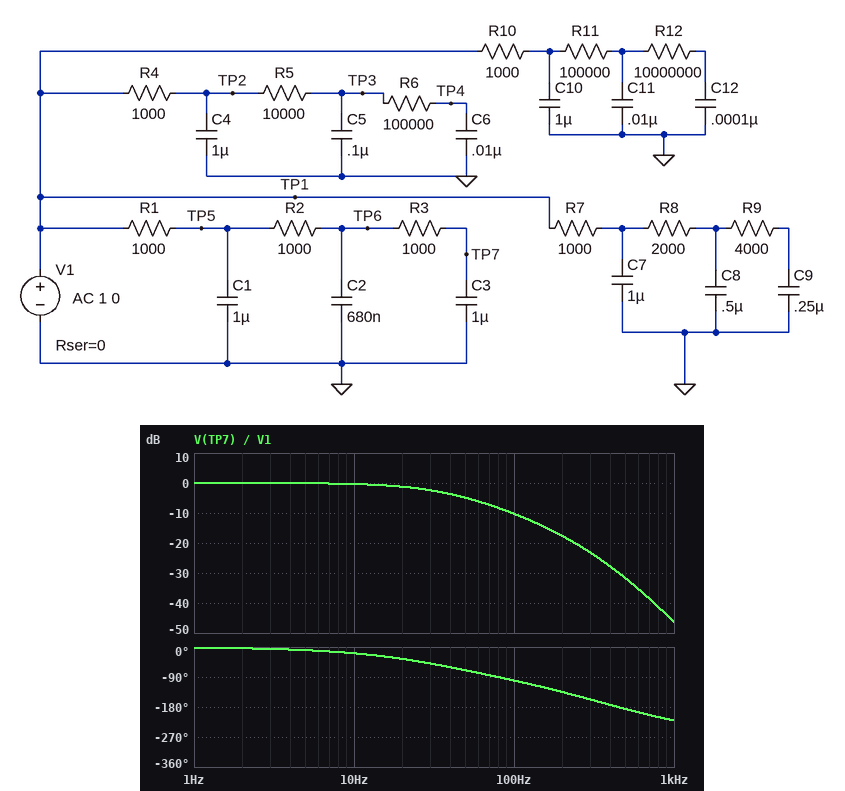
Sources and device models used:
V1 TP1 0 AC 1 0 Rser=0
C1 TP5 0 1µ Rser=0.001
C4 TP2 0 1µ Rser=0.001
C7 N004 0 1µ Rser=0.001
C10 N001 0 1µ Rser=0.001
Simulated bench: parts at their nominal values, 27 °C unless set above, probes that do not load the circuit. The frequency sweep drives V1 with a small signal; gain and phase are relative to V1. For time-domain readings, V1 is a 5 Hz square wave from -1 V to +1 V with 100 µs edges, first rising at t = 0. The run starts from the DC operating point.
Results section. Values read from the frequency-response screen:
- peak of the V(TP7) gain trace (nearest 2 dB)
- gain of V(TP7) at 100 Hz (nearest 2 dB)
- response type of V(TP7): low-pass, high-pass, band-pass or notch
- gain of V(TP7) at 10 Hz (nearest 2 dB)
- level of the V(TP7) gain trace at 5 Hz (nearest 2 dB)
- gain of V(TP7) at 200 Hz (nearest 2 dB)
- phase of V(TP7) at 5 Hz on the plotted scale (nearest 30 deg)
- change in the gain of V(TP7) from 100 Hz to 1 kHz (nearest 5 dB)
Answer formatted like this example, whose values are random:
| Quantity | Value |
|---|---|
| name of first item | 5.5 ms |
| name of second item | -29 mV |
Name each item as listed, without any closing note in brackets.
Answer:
| Quantity | Value |
|---|---|
| peak of the V(TP7) gain trace | 0 dB |
| gain of V(TP7) at 100 Hz | -10 dB |
| response type of V(TP7): low-pass, high-pass, band-pass or notch | low-pass |
| gain of V(TP7) at 10 Hz | 0 dB |
| level of the V(TP7) gain trace at 5 Hz | 0 dB |
| gain of V(TP7) at 200 Hz | -18 dB |
| phase of V(TP7) at 5 Hz on the plotted scale | 0 deg |
| change in the gain of V(TP7) from 100 Hz to 1 kHz | -35 dB |
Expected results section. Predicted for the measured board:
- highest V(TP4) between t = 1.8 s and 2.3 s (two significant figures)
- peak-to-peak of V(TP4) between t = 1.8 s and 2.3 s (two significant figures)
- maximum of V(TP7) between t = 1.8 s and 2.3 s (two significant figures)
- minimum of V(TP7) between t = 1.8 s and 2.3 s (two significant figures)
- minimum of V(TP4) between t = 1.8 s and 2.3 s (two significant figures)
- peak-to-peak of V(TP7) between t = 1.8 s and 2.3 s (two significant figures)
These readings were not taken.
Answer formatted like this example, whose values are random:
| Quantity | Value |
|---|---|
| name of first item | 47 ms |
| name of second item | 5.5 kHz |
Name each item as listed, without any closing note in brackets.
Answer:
| Quantity | Value |
|---|---|
| highest V(TP4) between t = 1.8 s and 2.3 s | 1.0 V |
| peak-to-peak of V(TP4) between t = 1.8 s and 2.3 s | 2.0 V |
| maximum of V(TP7) between t = 1.8 s and 2.3 s | 1.0 V |
| minimum of V(TP7) between t = 1.8 s and 2.3 s | -1.0 V |
| minimum of V(TP4) between t = 1.8 s and 2.3 s | -1.0 V |
| peak-to-peak of V(TP7) between t = 1.8 s and 2.3 s | 2.0 V |
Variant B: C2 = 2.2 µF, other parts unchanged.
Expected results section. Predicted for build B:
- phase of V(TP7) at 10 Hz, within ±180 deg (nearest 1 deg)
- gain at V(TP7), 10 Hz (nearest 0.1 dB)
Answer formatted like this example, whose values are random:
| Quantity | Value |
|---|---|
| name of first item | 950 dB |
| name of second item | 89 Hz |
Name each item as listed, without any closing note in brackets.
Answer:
| Quantity | Value |
|---|---|
| phase of V(TP7) at 10 Hz, within ±180 deg | -29 deg |
| gain at V(TP7), 10 Hz | -0.8 dB |
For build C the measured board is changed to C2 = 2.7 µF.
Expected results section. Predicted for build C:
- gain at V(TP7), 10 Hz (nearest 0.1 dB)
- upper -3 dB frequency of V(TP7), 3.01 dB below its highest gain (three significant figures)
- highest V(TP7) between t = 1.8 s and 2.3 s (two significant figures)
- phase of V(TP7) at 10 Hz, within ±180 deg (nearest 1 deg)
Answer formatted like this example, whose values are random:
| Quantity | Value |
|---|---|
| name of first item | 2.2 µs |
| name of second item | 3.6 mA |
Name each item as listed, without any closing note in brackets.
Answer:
| Quantity | Value |
|---|---|
| gain at V(TP7), 10 Hz | -1.0 dB |
| upper -3 dB frequency of V(TP7), 3.01 dB below its highest gain | 19.2 Hz |
| highest V(TP7) between t = 1.8 s and 2.3 s | 1.0 V |
| phase of V(TP7) at 10 Hz, within ±180 deg | -32 deg |
